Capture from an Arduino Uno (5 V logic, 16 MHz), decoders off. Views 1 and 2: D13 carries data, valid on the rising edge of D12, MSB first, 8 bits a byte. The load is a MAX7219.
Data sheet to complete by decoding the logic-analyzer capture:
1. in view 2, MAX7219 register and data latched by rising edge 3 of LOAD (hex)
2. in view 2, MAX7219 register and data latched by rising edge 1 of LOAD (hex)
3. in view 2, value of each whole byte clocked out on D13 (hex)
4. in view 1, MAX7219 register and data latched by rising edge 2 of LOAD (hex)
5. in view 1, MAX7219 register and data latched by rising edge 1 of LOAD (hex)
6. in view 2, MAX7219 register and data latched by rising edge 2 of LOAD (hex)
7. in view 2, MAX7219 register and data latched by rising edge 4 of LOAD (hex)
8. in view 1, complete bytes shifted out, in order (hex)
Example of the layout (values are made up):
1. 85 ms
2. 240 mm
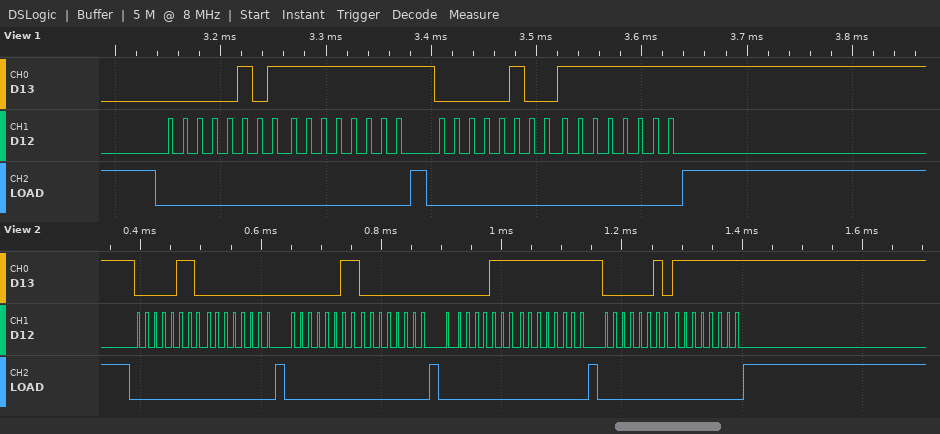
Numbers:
1. register 0x7, data 0xFF
2. register 0x6, data 0x00
3. 06 00 03 00 07 FF 02 FF
4. register 0x4, data 0xFF
5. register 0x5, data 0xFF
6. register 0x3, data 0x00
7. register 0x2, data 0xFF
8. 05 FF 04 FF
